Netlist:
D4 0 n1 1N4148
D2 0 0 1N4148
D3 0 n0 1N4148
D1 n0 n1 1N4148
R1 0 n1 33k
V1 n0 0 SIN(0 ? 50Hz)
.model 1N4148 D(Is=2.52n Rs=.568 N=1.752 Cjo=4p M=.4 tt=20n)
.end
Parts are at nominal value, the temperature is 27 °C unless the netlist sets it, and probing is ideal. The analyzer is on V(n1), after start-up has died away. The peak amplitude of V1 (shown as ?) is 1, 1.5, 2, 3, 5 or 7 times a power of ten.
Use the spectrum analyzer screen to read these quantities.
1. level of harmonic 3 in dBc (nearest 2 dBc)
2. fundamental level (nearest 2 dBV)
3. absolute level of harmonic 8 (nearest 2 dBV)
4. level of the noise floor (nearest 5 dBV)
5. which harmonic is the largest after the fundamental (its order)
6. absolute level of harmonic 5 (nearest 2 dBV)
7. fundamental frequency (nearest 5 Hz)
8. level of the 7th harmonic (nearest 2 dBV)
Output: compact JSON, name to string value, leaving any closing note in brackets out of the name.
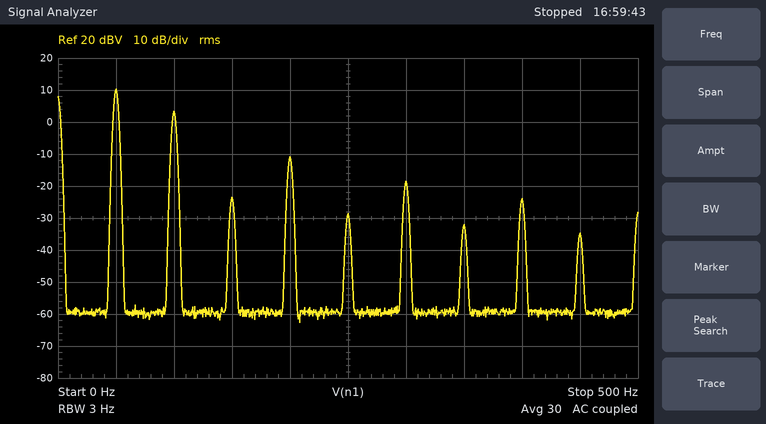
{"level of harmonic 3 in dBc": "-34 dBc", "fundamental level": "10 dBV", "absolute level of harmonic 8": "-24 dBV", "level of the noise floor": "-60 dBV", "which harmonic is the largest after the fundamental": "2", "absolute level of harmonic 5": "-28 dBV", "fundamental frequency": "50 Hz", "level of the 7th harmonic": "-32 dBV"}
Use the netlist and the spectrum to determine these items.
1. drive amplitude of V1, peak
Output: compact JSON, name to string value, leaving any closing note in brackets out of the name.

{"drive amplitude of V1, peak": "10 V"}
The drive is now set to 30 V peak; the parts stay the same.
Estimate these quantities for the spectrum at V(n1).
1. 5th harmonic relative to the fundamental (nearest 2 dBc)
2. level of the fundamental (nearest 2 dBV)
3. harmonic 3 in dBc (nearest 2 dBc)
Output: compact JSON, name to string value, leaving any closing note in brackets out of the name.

{"5th harmonic relative to the fundamental": "-48 dBc", "level of the fundamental": "20 dBV", "harmonic 3 in dBc": "-42 dBc"}
